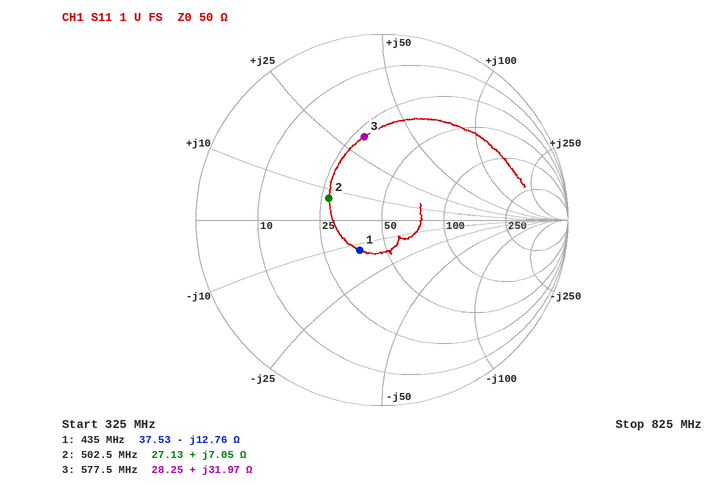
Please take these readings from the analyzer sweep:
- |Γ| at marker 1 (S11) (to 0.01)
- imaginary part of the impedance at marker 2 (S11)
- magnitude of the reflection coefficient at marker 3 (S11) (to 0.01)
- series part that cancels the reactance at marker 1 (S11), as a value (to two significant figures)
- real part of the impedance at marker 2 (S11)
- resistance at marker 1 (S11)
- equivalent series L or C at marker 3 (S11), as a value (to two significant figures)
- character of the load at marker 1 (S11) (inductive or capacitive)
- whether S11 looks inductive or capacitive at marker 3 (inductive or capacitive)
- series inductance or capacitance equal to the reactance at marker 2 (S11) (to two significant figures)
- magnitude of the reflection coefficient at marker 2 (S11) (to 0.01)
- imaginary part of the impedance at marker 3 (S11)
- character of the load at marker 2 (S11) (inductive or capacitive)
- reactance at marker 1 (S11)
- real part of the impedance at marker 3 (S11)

0.20
+7.05 Ω
0.46
4.7 nH
27.13 Ω
37.53 Ω
8.8 nH
capacitive
inductive
2.2 nH
0.31
+31.97 Ω
inductive
-12.76 Ω
28.25 Ω
